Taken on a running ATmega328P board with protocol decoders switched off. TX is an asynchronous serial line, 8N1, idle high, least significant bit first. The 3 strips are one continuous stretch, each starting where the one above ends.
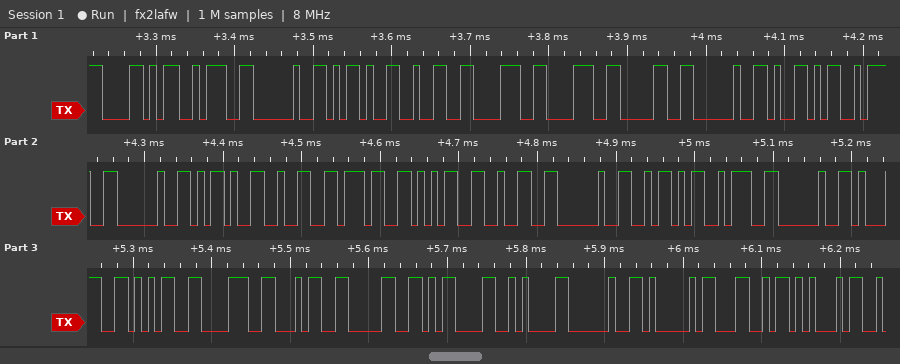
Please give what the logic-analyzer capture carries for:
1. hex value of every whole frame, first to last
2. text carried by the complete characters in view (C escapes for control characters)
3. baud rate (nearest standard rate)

58 3A 20 2D 32 38 38 30 20 59 3A 20 2D 32 37 35 32 20 5A 3A 20 31 35 38 34 30 0D 0A 20 41 4C 45
"X: -2880 Y: -2752 Z: 15840\r\n ALE"
115200 baud
